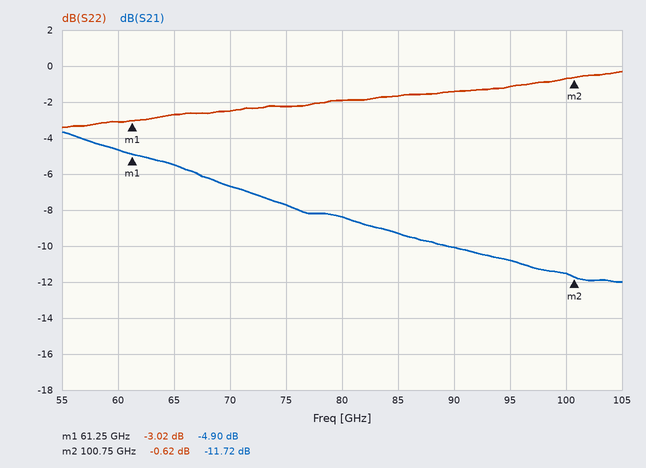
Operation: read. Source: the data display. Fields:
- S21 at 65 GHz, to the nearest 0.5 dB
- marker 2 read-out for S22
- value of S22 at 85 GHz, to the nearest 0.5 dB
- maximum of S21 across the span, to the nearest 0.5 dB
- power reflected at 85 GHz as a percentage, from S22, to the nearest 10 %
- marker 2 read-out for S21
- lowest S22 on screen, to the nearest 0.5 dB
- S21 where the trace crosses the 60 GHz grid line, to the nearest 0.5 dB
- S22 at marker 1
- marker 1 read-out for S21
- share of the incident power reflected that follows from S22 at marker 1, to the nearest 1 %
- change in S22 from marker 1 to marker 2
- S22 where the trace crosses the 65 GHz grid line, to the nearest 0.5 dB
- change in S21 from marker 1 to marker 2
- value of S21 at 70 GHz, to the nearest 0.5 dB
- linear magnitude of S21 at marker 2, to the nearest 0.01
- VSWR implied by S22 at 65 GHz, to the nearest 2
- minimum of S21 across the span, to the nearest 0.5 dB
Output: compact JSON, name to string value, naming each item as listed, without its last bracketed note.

{"S21 at 65 GHz, to the nearest 0.5 dB": "-5.5 dB", "marker 2 read-out for S22": "-0.62 dB", "value of S22 at 85 GHz, to the nearest 0.5 dB": "-1.5 dB", "maximum of S21 across the span, to the nearest 0.5 dB": "-3.5 dB", "power reflected at 85 GHz as a percentage, from S22, to the nearest 10 %": "70 %", "marker 2 read-out for S21": "-11.72 dB", "lowest S22 on screen, to the nearest 0.5 dB": "-3.5 dB", "S21 where the trace crosses the 60 GHz grid line, to the nearest 0.5 dB": "-4.5 dB", "S22 at marker 1": "-3.02 dB", "marker 1 read-out for S21": "-4.90 dB", "share of the incident power reflected that follows from S22 at marker 1, to the nearest 1 %": "50 %", "change in S22 from marker 1 to marker 2": "2.40 dB", "S22 where the trace crosses the 65 GHz grid line, to the nearest 0.5 dB": "-2.5 dB", "change in S21 from marker 1 to marker 2": "-6.82 dB", "value of S21 at 70 GHz, to the nearest 0.5 dB": "-6.5 dB", "linear magnitude of S21 at marker 2, to the nearest 0.01": "0.26", "VSWR implied by S22 at 65 GHz, to the nearest 2": "6", "minimum of S21 across the span, to the nearest 0.5 dB": "-12.0 dB"}
